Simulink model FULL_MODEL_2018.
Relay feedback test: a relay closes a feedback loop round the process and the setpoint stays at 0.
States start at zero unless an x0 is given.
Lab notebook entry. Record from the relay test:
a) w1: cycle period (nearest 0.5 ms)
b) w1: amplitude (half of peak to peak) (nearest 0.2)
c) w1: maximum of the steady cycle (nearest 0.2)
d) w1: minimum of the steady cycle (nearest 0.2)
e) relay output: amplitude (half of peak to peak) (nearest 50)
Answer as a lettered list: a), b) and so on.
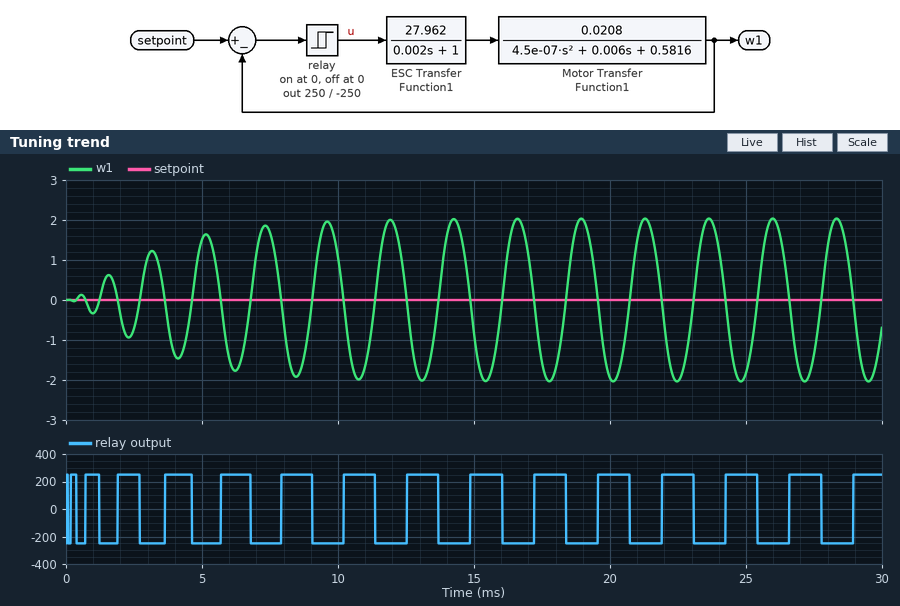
a) 2.5 ms
b) 2.0
c) 2.0
d) -2.0
e) 250
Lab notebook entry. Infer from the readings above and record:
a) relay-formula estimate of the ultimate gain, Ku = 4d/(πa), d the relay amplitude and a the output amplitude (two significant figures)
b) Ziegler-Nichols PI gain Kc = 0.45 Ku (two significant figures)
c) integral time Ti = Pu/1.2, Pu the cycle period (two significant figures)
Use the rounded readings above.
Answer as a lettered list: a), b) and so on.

a) 160
b) 72
c) 2.1 ms
